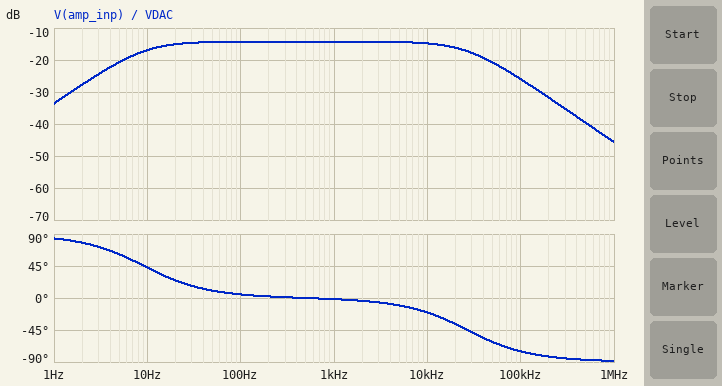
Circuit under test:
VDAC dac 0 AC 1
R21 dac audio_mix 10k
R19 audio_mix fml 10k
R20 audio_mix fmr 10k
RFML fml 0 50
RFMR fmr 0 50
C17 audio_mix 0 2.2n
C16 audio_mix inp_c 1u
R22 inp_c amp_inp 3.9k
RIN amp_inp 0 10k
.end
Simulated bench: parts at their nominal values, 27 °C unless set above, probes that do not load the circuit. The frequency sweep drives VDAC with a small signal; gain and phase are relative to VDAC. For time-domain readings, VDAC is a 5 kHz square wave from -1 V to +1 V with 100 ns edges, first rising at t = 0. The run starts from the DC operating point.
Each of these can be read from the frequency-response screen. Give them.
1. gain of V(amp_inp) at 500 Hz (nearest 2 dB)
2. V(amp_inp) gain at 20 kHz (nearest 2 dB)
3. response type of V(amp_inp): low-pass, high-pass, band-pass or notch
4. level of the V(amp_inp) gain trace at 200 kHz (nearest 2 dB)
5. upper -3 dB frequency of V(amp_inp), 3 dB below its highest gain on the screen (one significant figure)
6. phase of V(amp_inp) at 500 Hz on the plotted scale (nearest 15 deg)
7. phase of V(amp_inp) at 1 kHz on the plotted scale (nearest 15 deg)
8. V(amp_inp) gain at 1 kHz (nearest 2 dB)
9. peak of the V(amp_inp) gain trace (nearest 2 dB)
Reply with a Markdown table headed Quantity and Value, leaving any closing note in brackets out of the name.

| Quantity | Value |
|---|---|
| gain of V(amp_inp) at 500 Hz | -14 dB |
| V(amp_inp) gain at 20 kHz | -16 dB |
| response type of V(amp_inp): low-pass, high-pass, band-pass or notch | band-pass |
| level of the V(amp_inp) gain trace at 200 kHz | -32 dB |
| upper -3 dB frequency of V(amp_inp), 3 dB below its highest gain on the screen | 30 kHz |
| phase of V(amp_inp) at 500 Hz on the plotted scale | 0 deg |
| phase of V(amp_inp) at 1 kHz on the plotted scale | 0 deg |
| V(amp_inp) gain at 1 kHz | -14 dB |
| peak of the V(amp_inp) gain trace | -14 dB |
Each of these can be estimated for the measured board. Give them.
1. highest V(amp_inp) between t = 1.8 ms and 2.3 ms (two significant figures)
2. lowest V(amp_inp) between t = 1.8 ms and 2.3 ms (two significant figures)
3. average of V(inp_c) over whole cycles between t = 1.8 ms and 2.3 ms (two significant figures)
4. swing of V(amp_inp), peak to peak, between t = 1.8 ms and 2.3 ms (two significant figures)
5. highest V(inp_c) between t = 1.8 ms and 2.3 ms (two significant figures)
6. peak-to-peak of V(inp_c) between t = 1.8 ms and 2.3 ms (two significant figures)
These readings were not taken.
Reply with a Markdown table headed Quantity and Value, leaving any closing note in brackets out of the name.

| Quantity | Value |
|---|---|
| highest V(amp_inp) between t = 1.8 ms and 2.3 ms | 370 mV |
| lowest V(amp_inp) between t = 1.8 ms and 2.3 ms | -23 mV |
| average of V(inp_c) over whole cycles between t = 1.8 ms and 2.3 ms | 240 mV |
| swing of V(amp_inp), peak to peak, between t = 1.8 ms and 2.3 ms | 390 mV |
| highest V(inp_c) between t = 1.8 ms and 2.3 ms | 510 mV |
| peak-to-peak of V(inp_c) between t = 1.8 ms and 2.3 ms | 540 mV |
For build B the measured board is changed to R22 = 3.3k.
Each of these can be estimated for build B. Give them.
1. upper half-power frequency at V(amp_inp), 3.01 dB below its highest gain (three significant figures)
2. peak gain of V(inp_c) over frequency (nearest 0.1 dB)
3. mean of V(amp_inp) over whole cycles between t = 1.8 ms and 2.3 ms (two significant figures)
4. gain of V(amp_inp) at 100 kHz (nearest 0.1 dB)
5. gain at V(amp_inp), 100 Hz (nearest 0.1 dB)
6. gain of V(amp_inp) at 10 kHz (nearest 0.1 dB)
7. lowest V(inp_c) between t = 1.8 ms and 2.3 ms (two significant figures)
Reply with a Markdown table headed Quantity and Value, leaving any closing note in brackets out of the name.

| Quantity | Value |
|---|---|
| upper half-power frequency at V(amp_inp), 3.01 dB below its highest gain | 27.1 kHz |
| peak gain of V(inp_c) over frequency | -11.5 dB |
| mean of V(amp_inp) over whole cycles between t = 1.8 ms and 2.3 ms | 180 mV |
| gain of V(amp_inp) at 100 kHz | -25.6 dB |
| gain at V(amp_inp), 100 Hz | -14.0 dB |
| gain of V(amp_inp) at 10 kHz | -14.5 dB |
| lowest V(inp_c) between t = 1.8 ms and 2.3 ms | -33 mV |
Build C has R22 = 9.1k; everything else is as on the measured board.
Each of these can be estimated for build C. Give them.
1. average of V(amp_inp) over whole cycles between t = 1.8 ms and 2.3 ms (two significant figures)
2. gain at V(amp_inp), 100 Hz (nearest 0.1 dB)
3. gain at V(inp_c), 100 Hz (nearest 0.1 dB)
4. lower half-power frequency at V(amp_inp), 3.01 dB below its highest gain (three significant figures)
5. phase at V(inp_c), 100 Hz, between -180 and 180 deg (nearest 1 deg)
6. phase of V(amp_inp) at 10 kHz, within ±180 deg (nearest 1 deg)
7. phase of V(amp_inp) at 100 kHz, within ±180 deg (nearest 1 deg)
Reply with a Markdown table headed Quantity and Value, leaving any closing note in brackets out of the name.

| Quantity | Value |
|---|---|
| average of V(amp_inp) over whole cycles between t = 1.8 ms and 2.3 ms | 140 mV |
| gain at V(amp_inp), 100 Hz | -16.6 dB |
| gain at V(inp_c), 100 Hz | -10.9 dB |
| lower half-power frequency at V(amp_inp), 3.01 dB below its highest gain | 7.09 Hz |
| phase at V(inp_c), 100 Hz, between -180 and 180 deg | 4 deg |
| phase of V(amp_inp) at 10 kHz, within ±180 deg | -21 deg |
| phase of V(amp_inp) at 100 kHz, within ±180 deg | -76 deg |
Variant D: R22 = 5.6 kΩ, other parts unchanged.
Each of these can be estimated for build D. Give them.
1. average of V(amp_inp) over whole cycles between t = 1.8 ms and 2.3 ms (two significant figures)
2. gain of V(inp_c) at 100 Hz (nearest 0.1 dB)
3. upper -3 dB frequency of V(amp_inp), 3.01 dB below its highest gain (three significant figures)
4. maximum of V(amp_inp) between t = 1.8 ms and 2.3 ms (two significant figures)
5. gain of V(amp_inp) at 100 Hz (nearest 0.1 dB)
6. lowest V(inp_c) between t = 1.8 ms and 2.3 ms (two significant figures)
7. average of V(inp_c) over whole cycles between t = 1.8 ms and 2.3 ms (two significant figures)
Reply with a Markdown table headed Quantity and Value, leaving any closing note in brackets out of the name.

| Quantity | Value |
|---|---|
| average of V(amp_inp) over whole cycles between t = 1.8 ms and 2.3 ms | 160 mV |
| gain of V(inp_c) at 100 Hz | -11.2 dB |
| upper -3 dB frequency of V(amp_inp), 3.01 dB below its highest gain | 26.3 kHz |
| maximum of V(amp_inp) between t = 1.8 ms and 2.3 ms | 340 mV |
| gain of V(amp_inp) at 100 Hz | -15.1 dB |
| lowest V(inp_c) between t = 1.8 ms and 2.3 ms | -30 mV |
| average of V(inp_c) over whole cycles between t = 1.8 ms and 2.3 ms | 250 mV |
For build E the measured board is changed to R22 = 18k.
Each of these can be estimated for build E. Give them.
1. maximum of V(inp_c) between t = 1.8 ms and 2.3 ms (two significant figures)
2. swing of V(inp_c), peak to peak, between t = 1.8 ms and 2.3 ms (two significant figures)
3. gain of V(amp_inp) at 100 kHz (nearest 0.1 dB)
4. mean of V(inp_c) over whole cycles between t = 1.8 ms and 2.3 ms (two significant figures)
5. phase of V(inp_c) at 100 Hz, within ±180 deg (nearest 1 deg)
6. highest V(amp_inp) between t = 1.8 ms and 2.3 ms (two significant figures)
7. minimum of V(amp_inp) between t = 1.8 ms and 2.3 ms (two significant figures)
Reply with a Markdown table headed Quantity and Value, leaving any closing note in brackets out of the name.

| Quantity | Value |
|---|---|
| maximum of V(inp_c) between t = 1.8 ms and 2.3 ms | 580 mV |
| swing of V(inp_c), peak to peak, between t = 1.8 ms and 2.3 ms | 600 mV |
| gain of V(amp_inp) at 100 kHz | -32.0 dB |
| mean of V(inp_c) over whole cycles between t = 1.8 ms and 2.3 ms | 280 mV |
| phase of V(inp_c) at 100 Hz, within ±180 deg | 3 deg |
| highest V(amp_inp) between t = 1.8 ms and 2.3 ms | 210 mV |
| minimum of V(amp_inp) between t = 1.8 ms and 2.3 ms | -7.2 mV |
